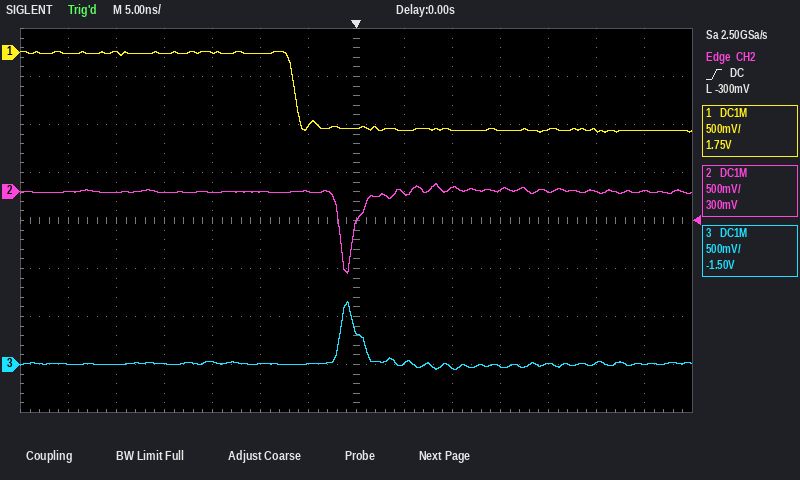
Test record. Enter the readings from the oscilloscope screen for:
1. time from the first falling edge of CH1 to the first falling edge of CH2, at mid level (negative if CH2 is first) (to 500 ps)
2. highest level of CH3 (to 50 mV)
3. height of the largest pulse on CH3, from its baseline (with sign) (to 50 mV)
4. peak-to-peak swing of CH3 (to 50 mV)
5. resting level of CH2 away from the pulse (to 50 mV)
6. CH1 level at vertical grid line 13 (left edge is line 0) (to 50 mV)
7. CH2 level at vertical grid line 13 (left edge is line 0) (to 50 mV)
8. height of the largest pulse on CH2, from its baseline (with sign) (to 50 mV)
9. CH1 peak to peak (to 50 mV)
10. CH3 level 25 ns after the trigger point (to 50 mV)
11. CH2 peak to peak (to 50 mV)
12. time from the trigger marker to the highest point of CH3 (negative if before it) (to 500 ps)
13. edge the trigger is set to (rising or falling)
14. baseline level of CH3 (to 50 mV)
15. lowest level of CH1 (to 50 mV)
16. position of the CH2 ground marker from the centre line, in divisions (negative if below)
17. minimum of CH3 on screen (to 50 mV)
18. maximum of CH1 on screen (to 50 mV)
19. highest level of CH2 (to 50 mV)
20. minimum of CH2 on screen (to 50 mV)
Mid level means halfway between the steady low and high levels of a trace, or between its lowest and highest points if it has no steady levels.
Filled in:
+4.5 ns
650 mV
+650 mV
700 mV
0 mV
-800 mV
0 mV
-850 mV
850 mV
0 mV
950 mV
-1.0 ns
rising
0 mV
-850 mV
+0.6 div
-50 mV
0 mV
100 mV
-850 mV
